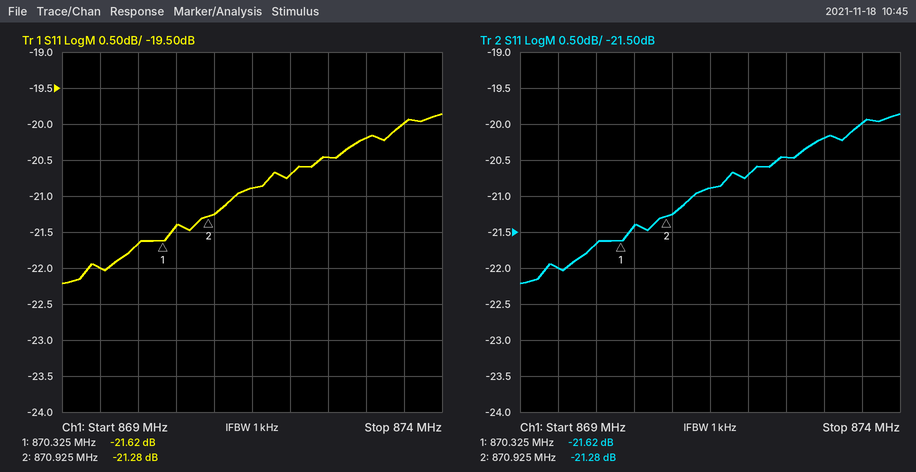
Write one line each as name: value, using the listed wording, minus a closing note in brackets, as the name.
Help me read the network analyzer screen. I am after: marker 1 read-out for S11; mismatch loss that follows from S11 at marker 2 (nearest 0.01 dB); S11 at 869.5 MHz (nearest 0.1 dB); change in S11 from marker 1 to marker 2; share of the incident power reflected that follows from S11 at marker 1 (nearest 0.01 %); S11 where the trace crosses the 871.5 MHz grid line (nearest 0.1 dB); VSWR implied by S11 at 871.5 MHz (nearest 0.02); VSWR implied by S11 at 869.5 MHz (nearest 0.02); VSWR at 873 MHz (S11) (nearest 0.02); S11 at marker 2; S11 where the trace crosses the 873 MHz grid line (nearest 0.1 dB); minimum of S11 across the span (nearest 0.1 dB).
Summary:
marker 1 read-out for S11: -21.62 dB
mismatch loss that follows from S11 at marker 2: 0.03 dB
S11 at 869.5 MHz: -22.0 dB
change in S11 from marker 1 to marker 2: 0.34 dB
share of the incident power reflected that follows from S11 at marker 1: 0.69 %
S11 where the trace crosses the 871.5 MHz grid line: -20.9 dB
VSWR implied by S11 at 871.5 MHz: 1.20
VSWR implied by S11 at 869.5 MHz: 1.18
VSWR at 873 MHz (S11): 1.22
S11 at marker 2: -21.28 dB
S11 where the trace crosses the 873 MHz grid line: -20.2 dB
minimum of S11 across the span: -22.2 dB
